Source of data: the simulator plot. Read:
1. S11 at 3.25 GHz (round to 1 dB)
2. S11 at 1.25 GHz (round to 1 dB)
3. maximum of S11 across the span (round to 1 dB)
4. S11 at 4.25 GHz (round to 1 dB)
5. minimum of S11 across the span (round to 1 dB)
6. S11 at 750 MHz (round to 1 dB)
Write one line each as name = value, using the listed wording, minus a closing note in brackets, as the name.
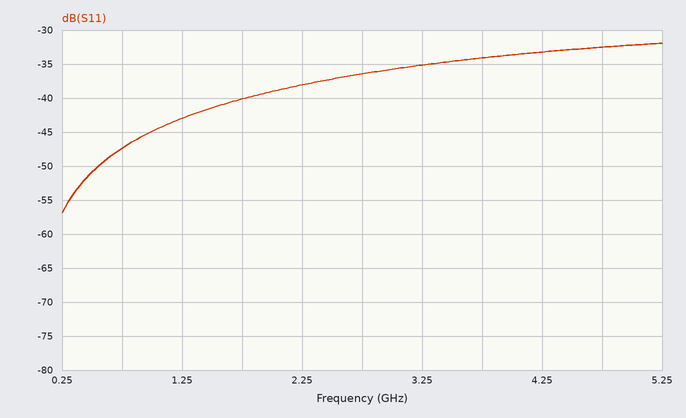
S11 at 3.25 GHz = -35 dB
S11 at 1.25 GHz = -43 dB
maximum of S11 across the span = -32 dB
S11 at 4.25 GHz = -33 dB
minimum of S11 across the span = -57 dB
S11 at 750 MHz = -47 dB
